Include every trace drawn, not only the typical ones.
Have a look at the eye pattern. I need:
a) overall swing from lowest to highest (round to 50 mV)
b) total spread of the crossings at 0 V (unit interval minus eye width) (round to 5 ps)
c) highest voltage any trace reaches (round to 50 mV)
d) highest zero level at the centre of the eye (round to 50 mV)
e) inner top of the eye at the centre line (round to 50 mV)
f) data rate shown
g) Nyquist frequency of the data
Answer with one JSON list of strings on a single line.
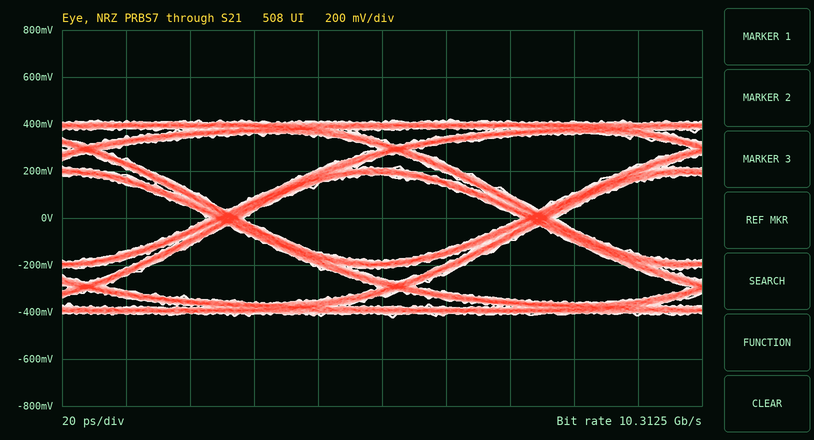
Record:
["850 mV", "10 ps", "400 mV", "-200 mV", "200 mV", "10.3125 Gb/s", "5.15625 GHz"]
